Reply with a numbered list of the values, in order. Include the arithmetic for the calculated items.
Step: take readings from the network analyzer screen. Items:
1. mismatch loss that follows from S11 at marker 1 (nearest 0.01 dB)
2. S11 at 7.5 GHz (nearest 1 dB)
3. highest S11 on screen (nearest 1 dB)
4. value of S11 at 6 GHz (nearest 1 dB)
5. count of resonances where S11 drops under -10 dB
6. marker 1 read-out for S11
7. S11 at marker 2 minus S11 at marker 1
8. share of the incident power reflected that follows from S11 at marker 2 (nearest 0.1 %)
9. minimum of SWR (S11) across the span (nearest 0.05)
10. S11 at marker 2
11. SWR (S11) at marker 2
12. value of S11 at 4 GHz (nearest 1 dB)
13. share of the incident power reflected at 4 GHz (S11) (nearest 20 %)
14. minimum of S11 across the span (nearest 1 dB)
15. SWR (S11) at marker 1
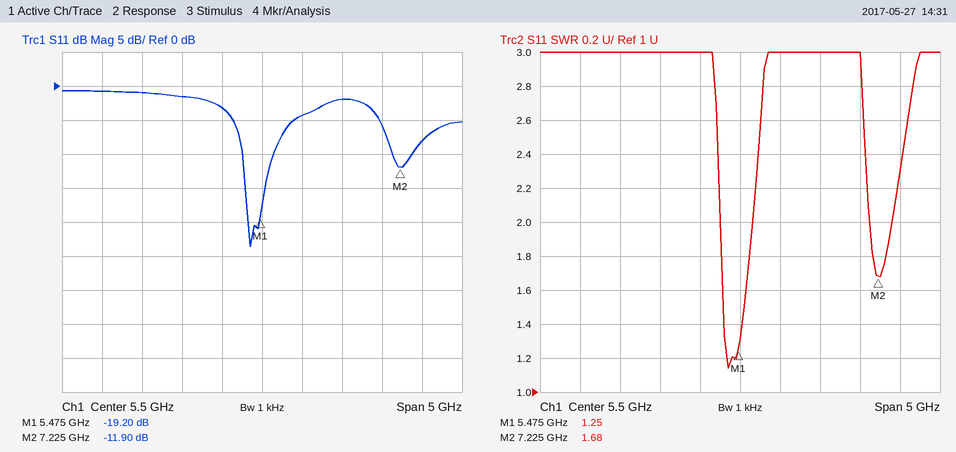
1. −10 log10(1 − 10^(-19.2/10)) ≈ 0.05 dB
2. -8 dB
3. -1 dB
4. -4 dB
5. 2
6. -19.20 dB
7. -11.9 − (-19.2) = 7.30 dB
8. 10^(-11.9/10) ≈ 6.5 %
9. 1.15
10. -11.90 dB
11. 1.68
12. -1 dB
13. 10^(-1/10) ≈ 79.4 %, so 80 % to the nearest 20 %
14. -24 dB
15. 1.25
